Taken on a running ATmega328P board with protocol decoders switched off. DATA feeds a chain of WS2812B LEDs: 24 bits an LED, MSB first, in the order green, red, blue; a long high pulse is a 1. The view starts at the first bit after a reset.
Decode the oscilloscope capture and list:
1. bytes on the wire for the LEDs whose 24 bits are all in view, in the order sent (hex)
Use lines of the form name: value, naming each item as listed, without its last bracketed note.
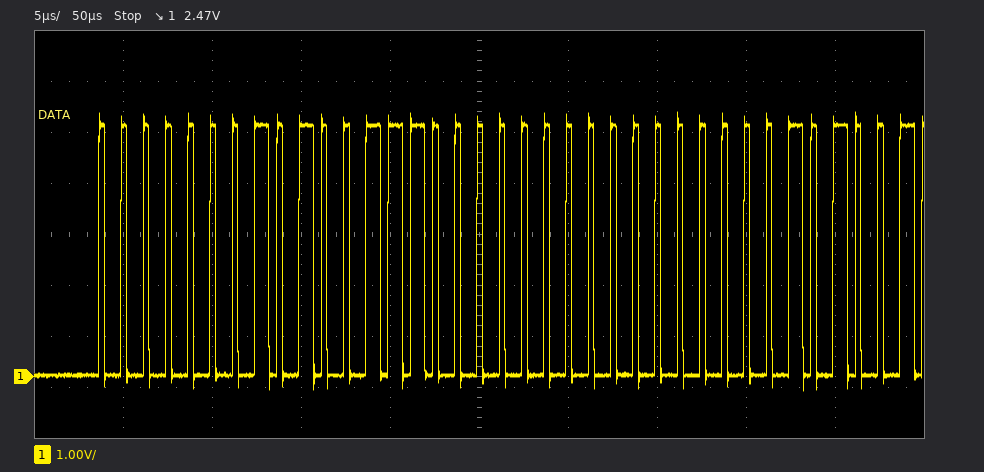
bytes on the wire for the LEDs whose 24 bits are all in view, in the order sent: 01 4E 00
